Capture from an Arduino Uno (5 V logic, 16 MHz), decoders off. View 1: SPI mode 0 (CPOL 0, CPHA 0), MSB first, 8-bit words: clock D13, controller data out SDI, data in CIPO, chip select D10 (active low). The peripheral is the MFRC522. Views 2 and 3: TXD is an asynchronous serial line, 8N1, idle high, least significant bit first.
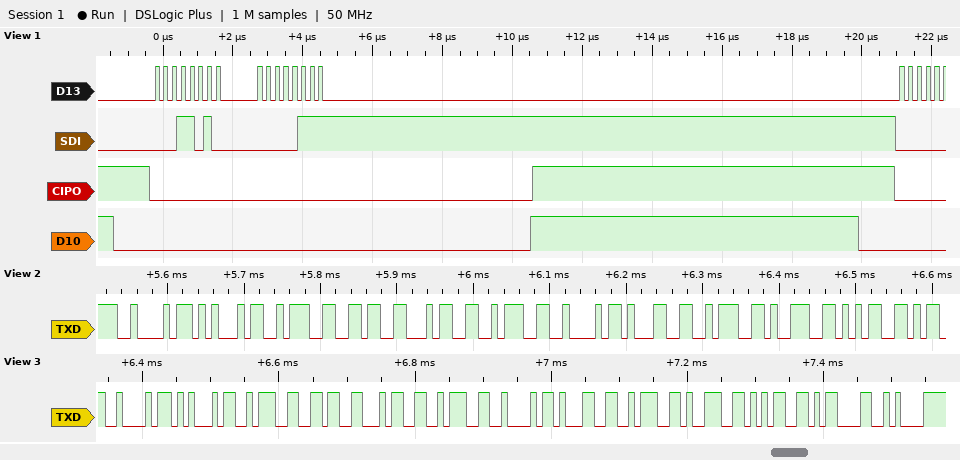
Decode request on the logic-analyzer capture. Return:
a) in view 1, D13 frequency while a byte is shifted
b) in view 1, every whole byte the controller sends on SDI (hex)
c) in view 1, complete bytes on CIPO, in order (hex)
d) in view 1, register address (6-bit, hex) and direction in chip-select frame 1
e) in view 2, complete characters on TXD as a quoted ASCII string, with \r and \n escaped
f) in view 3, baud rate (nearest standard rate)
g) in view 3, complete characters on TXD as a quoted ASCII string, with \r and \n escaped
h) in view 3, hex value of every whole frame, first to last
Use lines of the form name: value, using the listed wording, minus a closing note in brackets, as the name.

in view 1, D13 frequency while a byte is shifted: 4 MHz
in view 1, every whole byte the controller sends on SDI: 1A 07
in view 1, complete bytes on CIPO, in order: 00 00
in view 1, register address (6-bit, hex) and direction in chip-select frame 1: 0x0D write
in view 2, complete characters on TXD as a quoted ASCII string, with \r and \n escaped: "BE:64:B1:95"
in view 3, baud rate: 115200 baud
in view 3, complete characters on TXD as a quoted ASCII string, with \r and \n escaped: "BE:64:B1:95\r\n"
in view 3, hex value of every whole frame, first to last: 42 45 3A 36 34 3A 42 31 3A 39 35 0D 0A
